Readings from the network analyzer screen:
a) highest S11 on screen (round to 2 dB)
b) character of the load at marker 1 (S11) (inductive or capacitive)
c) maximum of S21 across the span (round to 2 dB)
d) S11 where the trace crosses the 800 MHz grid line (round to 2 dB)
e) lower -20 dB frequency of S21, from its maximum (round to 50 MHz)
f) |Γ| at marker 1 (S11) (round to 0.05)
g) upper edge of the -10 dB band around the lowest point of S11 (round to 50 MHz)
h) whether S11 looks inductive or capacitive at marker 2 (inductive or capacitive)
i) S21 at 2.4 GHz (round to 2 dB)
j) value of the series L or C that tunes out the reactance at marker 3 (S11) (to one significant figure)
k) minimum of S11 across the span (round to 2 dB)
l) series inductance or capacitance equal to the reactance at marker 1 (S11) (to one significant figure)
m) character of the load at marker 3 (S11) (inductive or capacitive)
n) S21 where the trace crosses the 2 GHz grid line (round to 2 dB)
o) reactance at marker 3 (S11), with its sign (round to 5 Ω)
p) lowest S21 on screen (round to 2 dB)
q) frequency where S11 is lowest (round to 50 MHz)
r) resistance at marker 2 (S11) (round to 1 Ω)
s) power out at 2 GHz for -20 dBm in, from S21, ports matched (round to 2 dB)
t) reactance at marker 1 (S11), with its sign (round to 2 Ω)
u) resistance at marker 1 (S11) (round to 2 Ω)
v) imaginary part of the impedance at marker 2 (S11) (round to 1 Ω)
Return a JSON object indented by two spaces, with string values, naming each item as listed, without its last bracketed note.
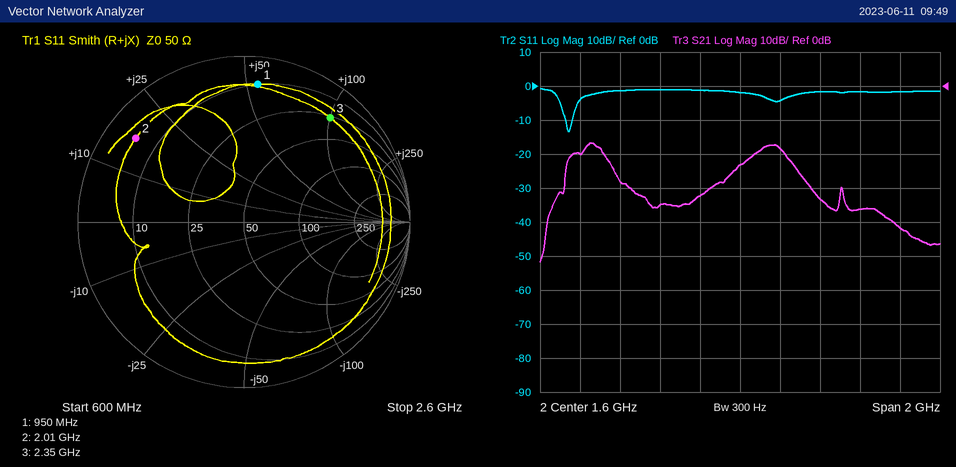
{
  "highest S11 on screen": "0 dB",
  "character of the load at marker 1 (S11)": "inductive",
  "maximum of S21 across the span": "-16 dB",
  "S11 where the trace crosses the 800 MHz grid line": "-4 dB",
  "lower -20 dB frequency of S21, from its maximum": "650 MHz",
  "|Γ| at marker 1 (S11)": "0.85",
  "upper edge of the -10 dB band around the lowest point of S11": "750 MHz",
  "whether S11 looks inductive or capacitive at marker 2": "inductive",
  "S21 at 2.4 GHz": "-42 dB",
  "value of the series L or C that tunes out the reactance at marker 3 (S11)": "700 fF",
  "minimum of S11 across the span": "-14 dB",
  "series inductance or capacitance equal to the reactance at marker 1 (S11)": "9 nH",
  "character of the load at marker 3 (S11)": "inductive",
  "S21 where the trace crosses the 2 GHz grid line": "-34 dB",
  "reactance at marker 3 (S11), with its sign": "+100 Ω",
  "lowest S21 on screen": "-52 dB",
  "frequency where S11 is lowest": "750 MHz",
  "resistance at marker 2 (S11)": "5 Ω",
  "power out at 2 GHz for -20 dBm in, from S21, ports matched": "-54 dBm",
  "reactance at marker 1 (S11), with its sign": "+54 Ω",
  "resistance at marker 1 (S11)": "10 Ω",
  "imaginary part of the impedance at marker 2 (S11)": "+17 Ω"
}
